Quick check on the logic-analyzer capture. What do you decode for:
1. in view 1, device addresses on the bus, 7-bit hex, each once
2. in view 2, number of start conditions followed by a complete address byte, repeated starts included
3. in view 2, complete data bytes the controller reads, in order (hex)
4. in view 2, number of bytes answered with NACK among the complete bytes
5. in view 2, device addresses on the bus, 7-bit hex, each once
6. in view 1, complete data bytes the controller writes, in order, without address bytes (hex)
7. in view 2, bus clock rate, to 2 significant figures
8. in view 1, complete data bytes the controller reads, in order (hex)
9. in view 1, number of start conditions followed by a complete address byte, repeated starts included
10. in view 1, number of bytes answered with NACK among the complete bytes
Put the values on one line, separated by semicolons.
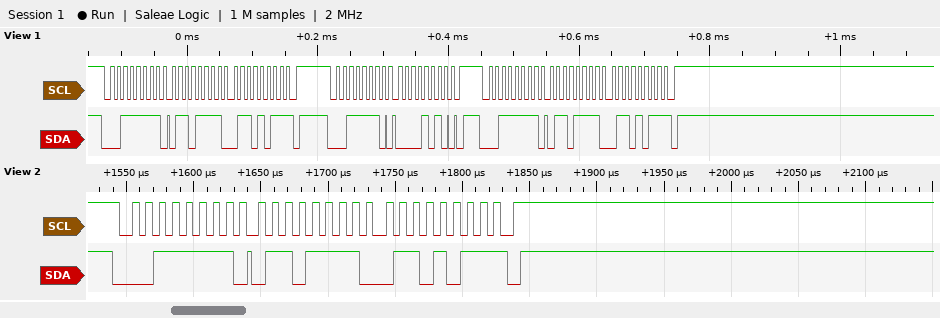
0x1F; 1; 6F 6B; 1; 0x1F; 0A; 100 kHz; 6F 6B 6F 6B; 3; 2
